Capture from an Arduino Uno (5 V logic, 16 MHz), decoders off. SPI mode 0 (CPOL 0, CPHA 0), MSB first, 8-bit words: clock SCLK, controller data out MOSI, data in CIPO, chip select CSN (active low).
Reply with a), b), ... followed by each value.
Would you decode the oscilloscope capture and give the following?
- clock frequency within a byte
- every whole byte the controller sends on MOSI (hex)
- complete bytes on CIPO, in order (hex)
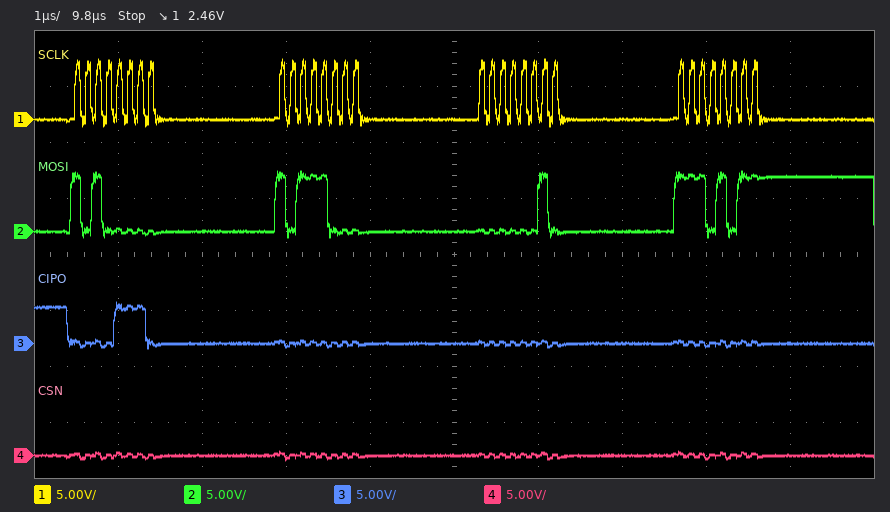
a) 8 MHz
b) 0xA0 0xB8 0x02 0xEB
c) 0x0E 0x00 0x00 0x00
